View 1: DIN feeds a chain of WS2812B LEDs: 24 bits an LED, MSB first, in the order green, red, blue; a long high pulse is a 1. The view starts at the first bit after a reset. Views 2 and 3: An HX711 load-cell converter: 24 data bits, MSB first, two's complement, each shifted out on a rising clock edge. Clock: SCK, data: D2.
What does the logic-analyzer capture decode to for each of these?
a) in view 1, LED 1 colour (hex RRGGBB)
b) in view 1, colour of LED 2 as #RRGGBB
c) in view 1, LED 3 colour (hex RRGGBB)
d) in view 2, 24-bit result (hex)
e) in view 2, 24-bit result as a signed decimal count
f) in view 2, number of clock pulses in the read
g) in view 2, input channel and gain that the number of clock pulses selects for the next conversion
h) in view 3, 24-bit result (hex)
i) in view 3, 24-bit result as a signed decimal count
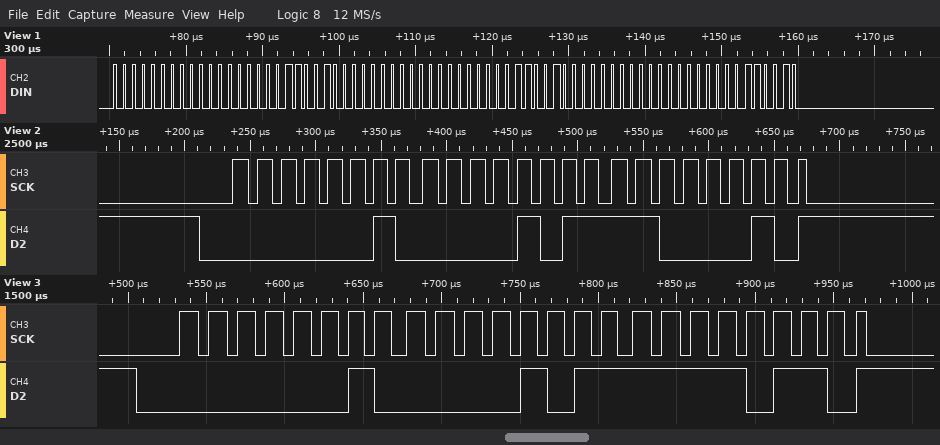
#000032
#000032
#000032
0x020BC2
134082
25
channel A, gain 128
0x020BF6
134134
